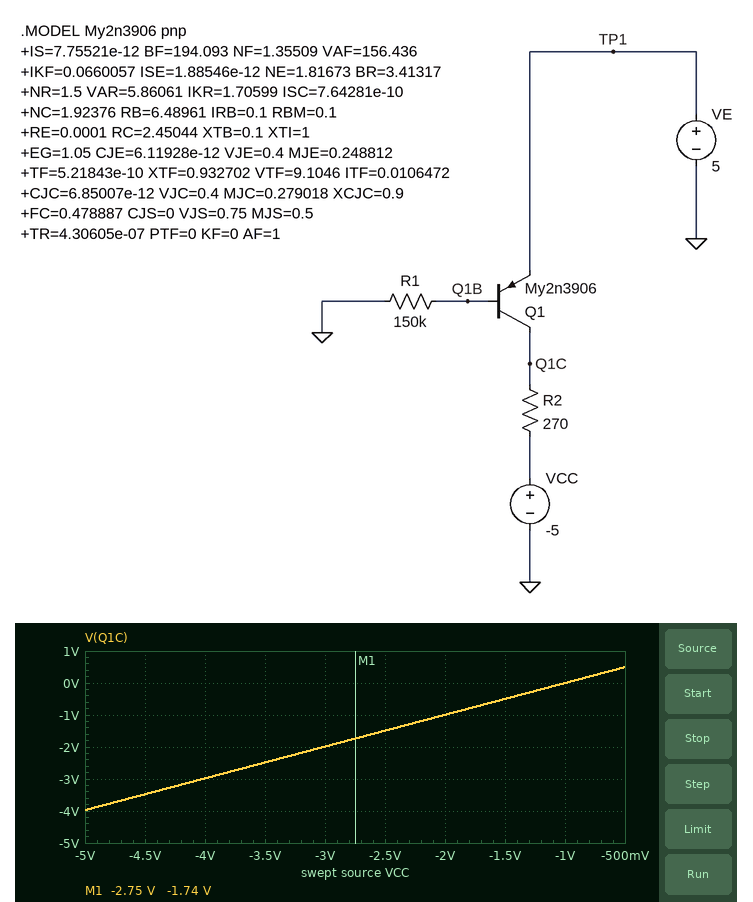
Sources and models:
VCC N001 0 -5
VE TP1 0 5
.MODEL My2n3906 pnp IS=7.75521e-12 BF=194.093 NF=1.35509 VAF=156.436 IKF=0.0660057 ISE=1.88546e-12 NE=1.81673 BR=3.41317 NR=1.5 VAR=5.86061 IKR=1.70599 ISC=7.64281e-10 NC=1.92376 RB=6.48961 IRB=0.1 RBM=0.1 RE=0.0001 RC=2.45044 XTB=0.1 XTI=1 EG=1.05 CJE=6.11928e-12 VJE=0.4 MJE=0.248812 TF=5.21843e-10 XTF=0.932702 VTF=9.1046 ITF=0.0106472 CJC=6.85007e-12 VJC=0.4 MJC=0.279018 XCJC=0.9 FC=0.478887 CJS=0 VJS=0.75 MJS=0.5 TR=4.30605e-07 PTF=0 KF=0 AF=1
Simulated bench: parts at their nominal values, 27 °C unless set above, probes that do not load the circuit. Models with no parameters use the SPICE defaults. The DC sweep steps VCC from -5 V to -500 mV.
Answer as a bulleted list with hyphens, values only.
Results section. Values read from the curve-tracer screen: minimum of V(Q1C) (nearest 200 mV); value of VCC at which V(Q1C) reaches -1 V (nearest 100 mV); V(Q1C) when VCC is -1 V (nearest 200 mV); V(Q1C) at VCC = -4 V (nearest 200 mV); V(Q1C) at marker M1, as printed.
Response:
- -4.0 V
- -2.0 V
- 0 V
- -3.0 V
- -1.74 V
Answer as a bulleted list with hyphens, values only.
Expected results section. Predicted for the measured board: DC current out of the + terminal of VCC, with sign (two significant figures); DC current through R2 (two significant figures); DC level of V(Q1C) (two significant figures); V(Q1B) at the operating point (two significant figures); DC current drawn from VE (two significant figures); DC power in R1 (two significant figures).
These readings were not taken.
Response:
- -3.8 mA
- 3.8 mA
- -4.0 V
- 4.3 V
- 3.8 mA
- 120 µW
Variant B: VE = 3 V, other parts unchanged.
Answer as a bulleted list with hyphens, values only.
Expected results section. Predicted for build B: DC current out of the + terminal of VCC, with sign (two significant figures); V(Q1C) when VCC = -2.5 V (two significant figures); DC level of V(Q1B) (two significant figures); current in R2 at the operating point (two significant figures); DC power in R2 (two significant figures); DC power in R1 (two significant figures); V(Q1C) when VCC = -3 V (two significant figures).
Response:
- -2.0 mA
- -2.0 V
- 2.3 V
- 2.0 mA
- 1.1 mW
- 36 µW
- -2.5 V
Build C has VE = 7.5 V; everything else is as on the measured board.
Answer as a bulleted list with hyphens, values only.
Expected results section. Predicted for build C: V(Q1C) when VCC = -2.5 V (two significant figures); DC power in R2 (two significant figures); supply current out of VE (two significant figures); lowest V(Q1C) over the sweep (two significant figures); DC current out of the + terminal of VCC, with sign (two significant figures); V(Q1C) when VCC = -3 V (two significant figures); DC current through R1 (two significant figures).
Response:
- -900 mV
- 9.8 mW
- 6.1 mA
- -3.4 V
- -6.0 mA
- -1.4 V
- 45 µA
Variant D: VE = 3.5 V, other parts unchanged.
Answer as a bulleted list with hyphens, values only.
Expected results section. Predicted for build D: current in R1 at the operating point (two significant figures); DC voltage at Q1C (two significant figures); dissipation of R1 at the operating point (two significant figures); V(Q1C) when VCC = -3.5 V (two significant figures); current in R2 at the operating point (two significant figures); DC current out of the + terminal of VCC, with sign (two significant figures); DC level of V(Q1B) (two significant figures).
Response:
- 19 µA
- -4.3 V
- 53 µW
- -2.8 V
- 2.5 mA
- -2.5 mA
- 2.8 V
